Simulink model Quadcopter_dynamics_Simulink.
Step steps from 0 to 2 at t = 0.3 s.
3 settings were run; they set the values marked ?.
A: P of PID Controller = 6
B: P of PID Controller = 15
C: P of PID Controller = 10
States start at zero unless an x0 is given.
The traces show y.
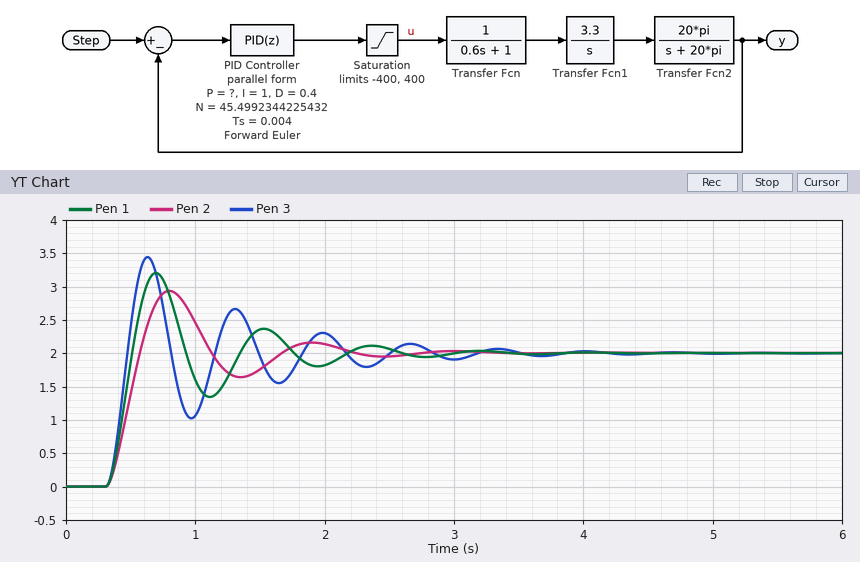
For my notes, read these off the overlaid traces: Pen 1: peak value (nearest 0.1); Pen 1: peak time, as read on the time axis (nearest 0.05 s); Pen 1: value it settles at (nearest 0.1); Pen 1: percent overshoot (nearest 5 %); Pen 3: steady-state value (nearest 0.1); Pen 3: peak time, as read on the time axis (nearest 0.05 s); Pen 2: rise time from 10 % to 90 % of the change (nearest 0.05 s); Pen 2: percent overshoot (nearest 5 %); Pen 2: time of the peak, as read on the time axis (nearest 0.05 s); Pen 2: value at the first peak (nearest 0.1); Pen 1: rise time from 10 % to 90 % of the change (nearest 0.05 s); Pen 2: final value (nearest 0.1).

3.2
0.70 s
2.0
60 %
2.0
0.65 s
0.20 s
45 %
0.80 s
2.9
0.15 s
2.0
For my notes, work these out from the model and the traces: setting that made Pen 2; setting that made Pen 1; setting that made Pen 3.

A
C
B
